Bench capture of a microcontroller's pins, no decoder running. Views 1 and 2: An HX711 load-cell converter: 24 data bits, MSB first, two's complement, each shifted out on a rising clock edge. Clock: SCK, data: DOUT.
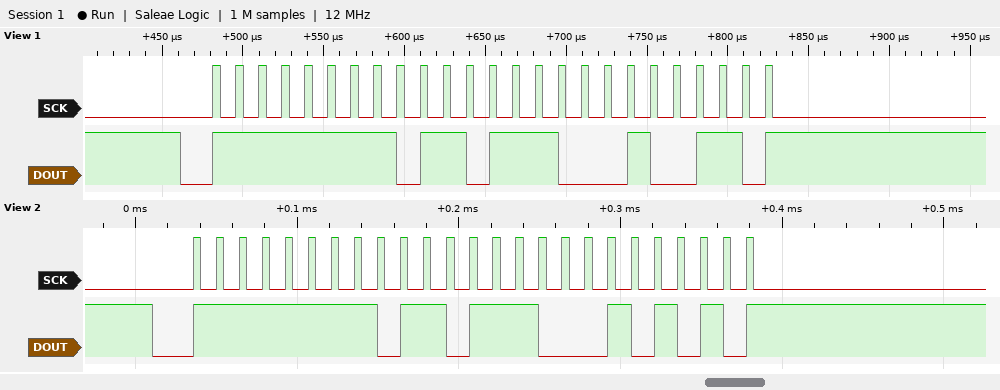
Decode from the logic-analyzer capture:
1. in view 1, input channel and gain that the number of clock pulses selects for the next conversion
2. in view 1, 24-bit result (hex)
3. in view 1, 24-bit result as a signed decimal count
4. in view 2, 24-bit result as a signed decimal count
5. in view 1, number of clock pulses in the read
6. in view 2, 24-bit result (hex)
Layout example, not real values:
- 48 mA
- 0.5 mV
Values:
- channel A, gain 128
- 0xFF6E26
- -37338
- -37334
- 25
- 0xFF6E2A
